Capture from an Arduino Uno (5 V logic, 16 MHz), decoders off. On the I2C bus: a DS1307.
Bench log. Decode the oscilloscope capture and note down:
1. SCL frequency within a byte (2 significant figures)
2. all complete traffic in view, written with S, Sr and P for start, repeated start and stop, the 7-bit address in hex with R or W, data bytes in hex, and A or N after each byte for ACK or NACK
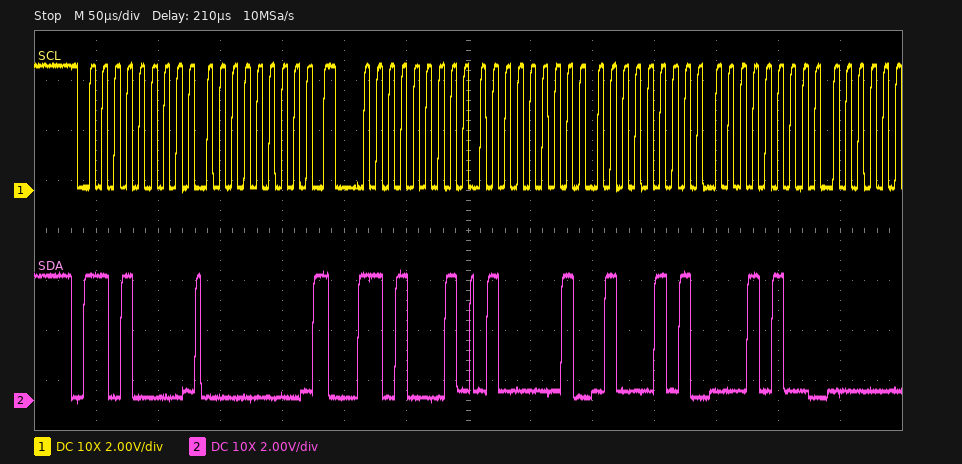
100 kHz
S 68W A 00 A Sr 68R A 41 A 45 A 14 A
